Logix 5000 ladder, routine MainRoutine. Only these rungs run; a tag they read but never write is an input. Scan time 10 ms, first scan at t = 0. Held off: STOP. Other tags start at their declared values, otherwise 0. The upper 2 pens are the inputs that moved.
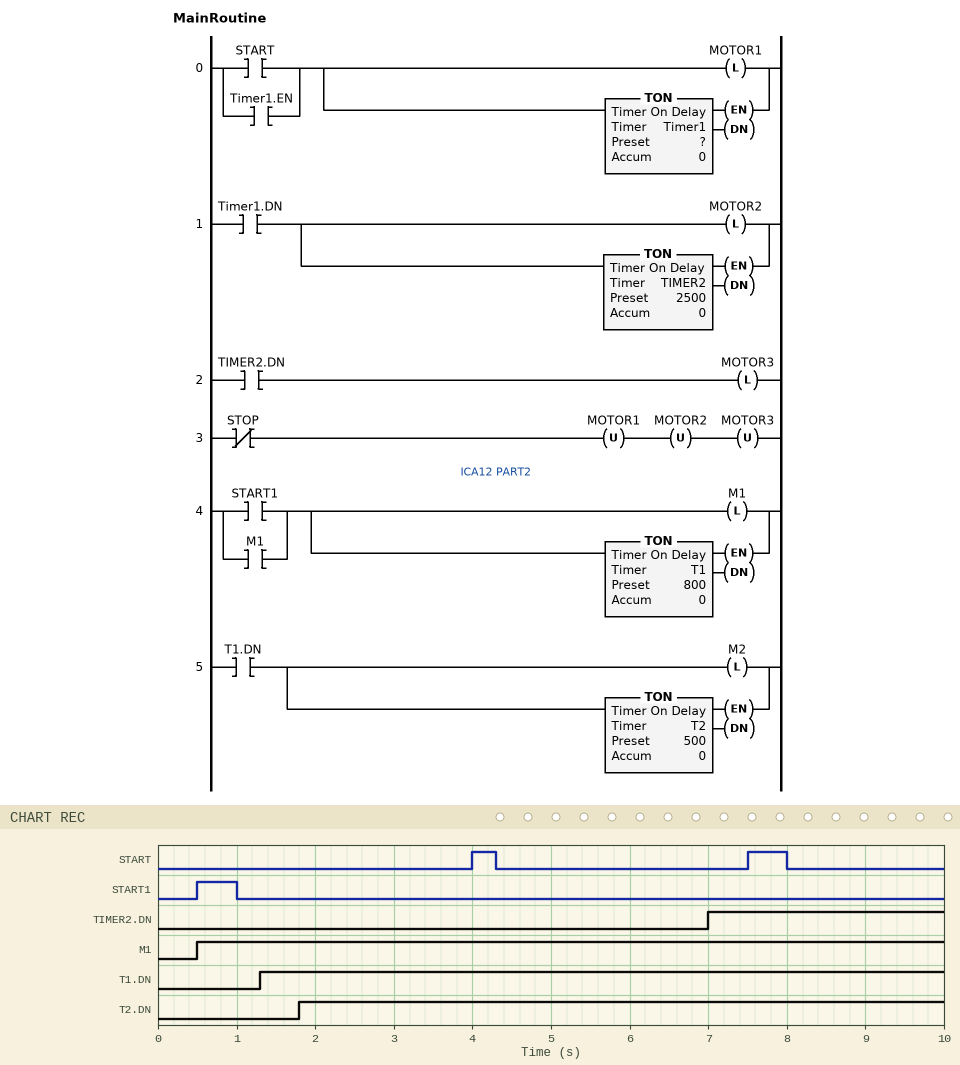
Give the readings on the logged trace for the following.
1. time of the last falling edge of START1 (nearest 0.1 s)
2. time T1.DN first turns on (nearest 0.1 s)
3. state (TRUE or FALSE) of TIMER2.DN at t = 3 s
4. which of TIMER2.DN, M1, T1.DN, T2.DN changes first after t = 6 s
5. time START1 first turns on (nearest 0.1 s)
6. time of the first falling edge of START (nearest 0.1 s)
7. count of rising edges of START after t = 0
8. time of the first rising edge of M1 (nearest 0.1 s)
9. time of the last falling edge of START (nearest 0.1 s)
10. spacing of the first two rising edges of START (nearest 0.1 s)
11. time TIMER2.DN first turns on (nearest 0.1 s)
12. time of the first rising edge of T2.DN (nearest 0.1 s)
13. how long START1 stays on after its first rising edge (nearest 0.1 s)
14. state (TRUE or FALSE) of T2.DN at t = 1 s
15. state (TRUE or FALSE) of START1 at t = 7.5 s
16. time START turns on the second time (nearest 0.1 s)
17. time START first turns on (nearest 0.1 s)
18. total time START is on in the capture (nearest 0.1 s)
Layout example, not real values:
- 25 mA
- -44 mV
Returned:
- 1.0 s
- 1.3 s
- FALSE
- TIMER2.DN
- 0.5 s
- 4.3 s
- 2
- 0.5 s
- 8.0 s
- 3.5 s
- 7.0 s
- 1.8 s
- 0.5 s
- FALSE
- FALSE
- 7.5 s
- 4.0 s
- 0.8 s
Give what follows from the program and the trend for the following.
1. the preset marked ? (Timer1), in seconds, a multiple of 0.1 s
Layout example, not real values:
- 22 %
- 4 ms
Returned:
- 0.5 s
